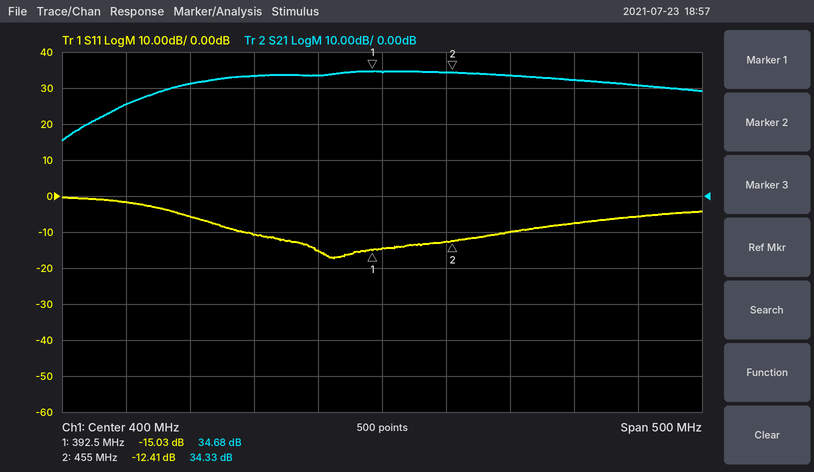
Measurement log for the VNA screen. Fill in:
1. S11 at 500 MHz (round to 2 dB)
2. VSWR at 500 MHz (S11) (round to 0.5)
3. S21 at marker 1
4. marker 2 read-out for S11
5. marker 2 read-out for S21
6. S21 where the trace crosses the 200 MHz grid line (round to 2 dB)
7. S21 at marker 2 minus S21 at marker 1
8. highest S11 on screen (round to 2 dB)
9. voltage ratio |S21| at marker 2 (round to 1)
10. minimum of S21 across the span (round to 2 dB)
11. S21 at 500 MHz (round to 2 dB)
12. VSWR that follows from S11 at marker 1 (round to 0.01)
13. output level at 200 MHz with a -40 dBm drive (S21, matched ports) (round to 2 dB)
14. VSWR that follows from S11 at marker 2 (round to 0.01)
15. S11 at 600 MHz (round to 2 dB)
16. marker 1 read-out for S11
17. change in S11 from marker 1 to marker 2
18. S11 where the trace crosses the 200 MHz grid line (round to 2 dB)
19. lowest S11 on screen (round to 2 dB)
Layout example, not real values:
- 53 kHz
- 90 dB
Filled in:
- -10 dB
- 2.0
- 34.68 dB
- -12.41 dB
- 34.33 dB
- 26 dB
- -0.35 dB
- 0 dB
- 52
- 16 dB
- 34 dB
- 1.43
- -14 dBm
- 1.63
- -6 dB
- -15.03 dB
- 2.62 dB
- -2 dB
- -18 dB
